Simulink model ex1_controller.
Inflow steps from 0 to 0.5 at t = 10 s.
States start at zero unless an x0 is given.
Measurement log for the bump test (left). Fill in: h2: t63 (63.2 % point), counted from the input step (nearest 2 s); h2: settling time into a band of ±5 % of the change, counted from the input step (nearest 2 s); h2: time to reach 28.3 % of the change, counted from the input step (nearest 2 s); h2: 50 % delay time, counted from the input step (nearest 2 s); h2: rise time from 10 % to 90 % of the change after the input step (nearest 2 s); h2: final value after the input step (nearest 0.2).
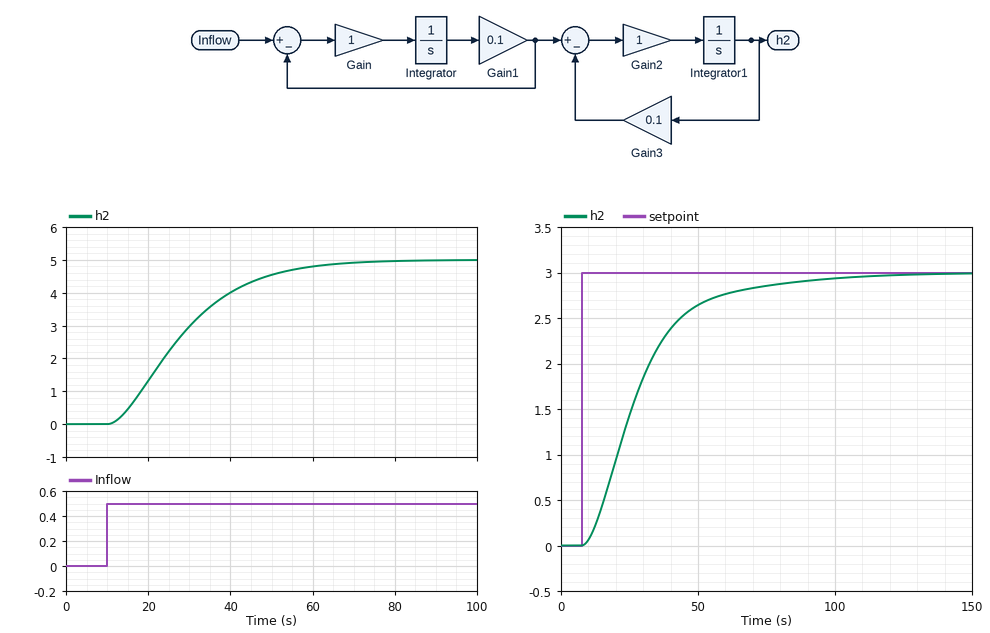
22 s
48 s
10 s
16 s
34 s
5.0
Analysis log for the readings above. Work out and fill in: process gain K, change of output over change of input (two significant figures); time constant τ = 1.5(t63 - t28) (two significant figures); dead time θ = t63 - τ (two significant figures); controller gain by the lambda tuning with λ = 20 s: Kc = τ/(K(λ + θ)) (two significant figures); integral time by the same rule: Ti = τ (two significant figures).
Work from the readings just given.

10
18 s
4.0 s
0.075
18 s
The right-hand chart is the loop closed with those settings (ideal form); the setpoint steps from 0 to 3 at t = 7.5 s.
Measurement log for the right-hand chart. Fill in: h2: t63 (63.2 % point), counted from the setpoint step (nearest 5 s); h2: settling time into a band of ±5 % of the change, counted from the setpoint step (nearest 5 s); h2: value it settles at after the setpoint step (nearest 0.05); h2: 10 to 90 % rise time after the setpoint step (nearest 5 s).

25 s
65 s
3.00
40 s
